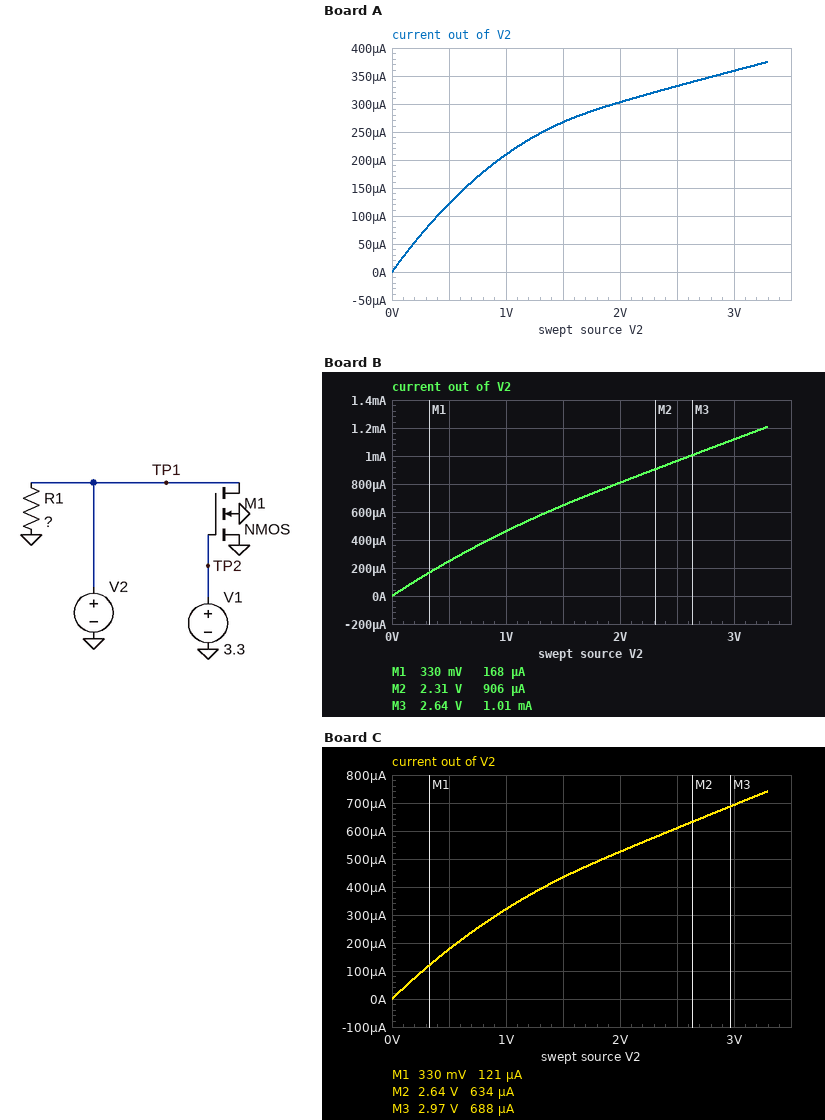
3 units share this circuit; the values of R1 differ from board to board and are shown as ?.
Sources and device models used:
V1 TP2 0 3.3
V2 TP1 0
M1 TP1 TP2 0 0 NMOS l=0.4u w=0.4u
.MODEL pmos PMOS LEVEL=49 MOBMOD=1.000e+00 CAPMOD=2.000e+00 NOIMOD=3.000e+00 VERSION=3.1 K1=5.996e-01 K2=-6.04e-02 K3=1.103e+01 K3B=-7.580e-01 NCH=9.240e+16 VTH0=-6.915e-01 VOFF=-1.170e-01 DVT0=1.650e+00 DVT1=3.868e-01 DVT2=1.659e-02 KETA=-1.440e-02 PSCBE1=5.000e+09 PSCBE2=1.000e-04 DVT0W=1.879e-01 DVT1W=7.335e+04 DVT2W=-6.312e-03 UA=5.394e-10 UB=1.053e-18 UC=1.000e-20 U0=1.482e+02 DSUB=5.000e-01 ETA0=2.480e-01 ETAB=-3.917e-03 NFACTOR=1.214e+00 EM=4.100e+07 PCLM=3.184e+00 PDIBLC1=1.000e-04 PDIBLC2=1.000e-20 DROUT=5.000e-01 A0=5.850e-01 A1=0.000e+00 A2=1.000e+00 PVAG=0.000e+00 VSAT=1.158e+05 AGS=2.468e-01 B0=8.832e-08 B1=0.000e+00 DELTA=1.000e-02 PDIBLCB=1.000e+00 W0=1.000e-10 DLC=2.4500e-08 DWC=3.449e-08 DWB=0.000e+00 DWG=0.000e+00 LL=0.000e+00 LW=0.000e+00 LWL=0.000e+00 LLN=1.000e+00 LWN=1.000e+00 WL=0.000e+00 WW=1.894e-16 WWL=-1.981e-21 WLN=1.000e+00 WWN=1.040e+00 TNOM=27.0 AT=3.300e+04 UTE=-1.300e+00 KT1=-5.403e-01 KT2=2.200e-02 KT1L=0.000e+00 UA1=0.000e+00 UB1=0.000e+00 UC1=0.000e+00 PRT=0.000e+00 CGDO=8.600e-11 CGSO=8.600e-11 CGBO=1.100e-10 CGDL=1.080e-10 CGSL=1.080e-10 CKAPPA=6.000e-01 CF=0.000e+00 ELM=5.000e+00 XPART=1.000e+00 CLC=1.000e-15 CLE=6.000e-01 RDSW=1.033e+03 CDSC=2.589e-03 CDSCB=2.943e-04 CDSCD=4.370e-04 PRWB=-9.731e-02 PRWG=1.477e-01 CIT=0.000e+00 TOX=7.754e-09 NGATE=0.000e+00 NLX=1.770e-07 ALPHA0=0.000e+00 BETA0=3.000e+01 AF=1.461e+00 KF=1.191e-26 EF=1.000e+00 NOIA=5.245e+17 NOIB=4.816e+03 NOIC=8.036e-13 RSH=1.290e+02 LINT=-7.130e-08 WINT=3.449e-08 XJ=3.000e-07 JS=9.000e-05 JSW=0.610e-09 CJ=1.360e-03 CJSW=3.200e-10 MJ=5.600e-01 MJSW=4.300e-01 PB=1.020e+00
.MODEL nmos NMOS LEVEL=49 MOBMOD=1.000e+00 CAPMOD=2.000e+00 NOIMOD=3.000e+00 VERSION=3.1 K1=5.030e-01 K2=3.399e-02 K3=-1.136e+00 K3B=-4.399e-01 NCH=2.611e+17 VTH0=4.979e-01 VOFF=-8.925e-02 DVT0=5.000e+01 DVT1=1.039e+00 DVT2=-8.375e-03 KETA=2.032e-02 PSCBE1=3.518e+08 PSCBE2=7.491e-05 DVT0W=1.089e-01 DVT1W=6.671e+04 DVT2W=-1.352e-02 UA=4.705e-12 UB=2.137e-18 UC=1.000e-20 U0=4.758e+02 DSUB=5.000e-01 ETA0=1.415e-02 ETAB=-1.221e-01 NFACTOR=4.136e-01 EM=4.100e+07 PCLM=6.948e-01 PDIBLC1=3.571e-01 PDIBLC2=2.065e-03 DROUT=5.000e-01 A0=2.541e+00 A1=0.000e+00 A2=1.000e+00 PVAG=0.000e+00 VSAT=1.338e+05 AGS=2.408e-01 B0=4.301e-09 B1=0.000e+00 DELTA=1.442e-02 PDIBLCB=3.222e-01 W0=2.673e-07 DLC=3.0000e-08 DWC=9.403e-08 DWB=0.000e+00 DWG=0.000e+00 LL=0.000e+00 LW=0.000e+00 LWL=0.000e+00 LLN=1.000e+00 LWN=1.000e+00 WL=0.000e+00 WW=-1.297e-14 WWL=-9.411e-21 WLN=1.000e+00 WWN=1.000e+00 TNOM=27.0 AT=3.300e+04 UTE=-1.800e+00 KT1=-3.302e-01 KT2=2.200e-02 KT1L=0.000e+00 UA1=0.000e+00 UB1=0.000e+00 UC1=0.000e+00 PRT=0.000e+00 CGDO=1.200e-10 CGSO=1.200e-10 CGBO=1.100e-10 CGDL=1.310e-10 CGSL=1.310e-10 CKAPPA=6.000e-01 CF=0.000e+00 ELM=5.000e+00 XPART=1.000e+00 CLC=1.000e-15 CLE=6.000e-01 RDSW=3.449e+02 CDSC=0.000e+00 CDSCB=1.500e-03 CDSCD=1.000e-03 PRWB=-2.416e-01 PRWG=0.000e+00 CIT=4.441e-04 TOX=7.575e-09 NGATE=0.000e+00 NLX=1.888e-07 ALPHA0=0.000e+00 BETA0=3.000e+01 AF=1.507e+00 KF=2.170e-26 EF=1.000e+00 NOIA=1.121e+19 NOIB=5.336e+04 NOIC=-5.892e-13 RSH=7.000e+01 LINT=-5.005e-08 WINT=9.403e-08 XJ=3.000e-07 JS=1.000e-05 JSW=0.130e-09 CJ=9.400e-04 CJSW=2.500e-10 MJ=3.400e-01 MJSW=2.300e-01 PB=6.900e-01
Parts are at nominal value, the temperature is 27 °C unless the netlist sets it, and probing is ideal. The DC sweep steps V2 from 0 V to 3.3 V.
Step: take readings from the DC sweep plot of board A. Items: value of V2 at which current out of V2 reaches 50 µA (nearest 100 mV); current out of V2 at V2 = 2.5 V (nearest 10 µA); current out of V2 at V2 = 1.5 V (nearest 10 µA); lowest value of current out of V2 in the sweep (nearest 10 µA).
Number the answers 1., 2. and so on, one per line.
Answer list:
1. 200 mV
2. 330 µA
3. 270 µA
4. 0 A
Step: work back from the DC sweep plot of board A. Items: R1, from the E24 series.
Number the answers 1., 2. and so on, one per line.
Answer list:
1. 20 kΩ
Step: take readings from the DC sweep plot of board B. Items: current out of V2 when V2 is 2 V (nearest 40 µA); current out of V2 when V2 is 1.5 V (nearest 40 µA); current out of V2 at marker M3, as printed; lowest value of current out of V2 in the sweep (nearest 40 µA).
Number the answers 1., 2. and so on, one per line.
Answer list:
1. 800 µA
2. 640 µA
3. 1.01 mA
4. 0 A
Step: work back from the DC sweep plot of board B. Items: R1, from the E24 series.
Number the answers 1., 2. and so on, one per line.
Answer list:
1. 3.3 kΩ
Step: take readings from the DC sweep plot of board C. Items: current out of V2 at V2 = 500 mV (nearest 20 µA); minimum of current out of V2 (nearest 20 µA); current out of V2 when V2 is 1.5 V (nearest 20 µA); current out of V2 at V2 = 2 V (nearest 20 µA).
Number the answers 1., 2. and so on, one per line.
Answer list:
1. 180 µA
2. 0 A
3. 440 µA
4. 520 µA
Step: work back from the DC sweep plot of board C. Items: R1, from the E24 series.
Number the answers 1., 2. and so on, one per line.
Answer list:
1. 6.2 kΩ
